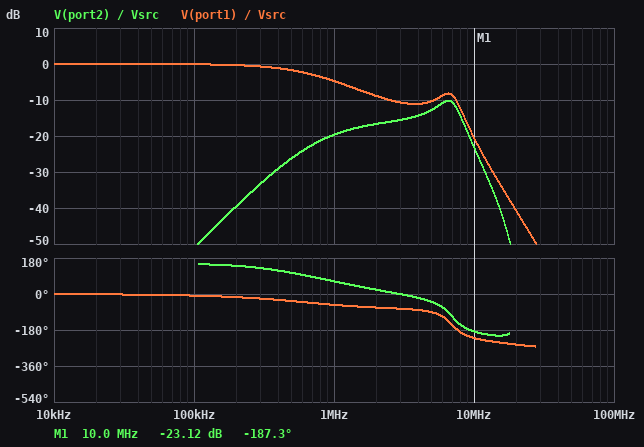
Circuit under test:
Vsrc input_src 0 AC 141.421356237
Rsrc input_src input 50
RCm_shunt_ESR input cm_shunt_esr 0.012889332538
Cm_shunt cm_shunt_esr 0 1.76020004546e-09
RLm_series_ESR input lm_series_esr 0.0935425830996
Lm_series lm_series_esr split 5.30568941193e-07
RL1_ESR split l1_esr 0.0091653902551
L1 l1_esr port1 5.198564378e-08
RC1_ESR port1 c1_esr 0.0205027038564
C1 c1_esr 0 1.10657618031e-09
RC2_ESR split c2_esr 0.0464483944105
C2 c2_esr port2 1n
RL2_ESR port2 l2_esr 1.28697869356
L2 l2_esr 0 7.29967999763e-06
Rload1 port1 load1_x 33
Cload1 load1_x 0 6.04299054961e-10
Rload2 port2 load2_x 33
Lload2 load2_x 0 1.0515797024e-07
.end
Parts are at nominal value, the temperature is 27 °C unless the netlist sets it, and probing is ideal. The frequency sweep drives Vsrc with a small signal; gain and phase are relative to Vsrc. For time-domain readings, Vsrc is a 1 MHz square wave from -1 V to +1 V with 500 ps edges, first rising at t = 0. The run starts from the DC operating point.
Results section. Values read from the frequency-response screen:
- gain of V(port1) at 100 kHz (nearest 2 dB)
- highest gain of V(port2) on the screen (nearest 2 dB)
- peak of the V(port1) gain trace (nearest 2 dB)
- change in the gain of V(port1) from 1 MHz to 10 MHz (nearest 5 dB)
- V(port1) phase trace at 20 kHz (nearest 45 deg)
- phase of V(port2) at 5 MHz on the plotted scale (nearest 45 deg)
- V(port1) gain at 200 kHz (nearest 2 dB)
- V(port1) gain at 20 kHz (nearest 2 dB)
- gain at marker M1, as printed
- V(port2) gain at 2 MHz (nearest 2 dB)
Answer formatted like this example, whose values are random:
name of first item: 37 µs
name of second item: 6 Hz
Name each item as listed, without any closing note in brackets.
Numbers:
gain of V(port1) at 100 kHz: 0 dB
highest gain of V(port2) on the screen: -10 dB
peak of the V(port1) gain trace: 0 dB
change in the gain of V(port1) from 1 MHz to 10 MHz: -15 dB
V(port1) phase trace at 20 kHz: 0 deg
phase of V(port2) at 5 MHz on the plotted scale: -45 deg
V(port1) gain at 200 kHz: 0 dB
V(port1) gain at 20 kHz: 0 dB
gain at marker M1, as printed: -23.12 dB
V(port2) gain at 2 MHz: -16 dB
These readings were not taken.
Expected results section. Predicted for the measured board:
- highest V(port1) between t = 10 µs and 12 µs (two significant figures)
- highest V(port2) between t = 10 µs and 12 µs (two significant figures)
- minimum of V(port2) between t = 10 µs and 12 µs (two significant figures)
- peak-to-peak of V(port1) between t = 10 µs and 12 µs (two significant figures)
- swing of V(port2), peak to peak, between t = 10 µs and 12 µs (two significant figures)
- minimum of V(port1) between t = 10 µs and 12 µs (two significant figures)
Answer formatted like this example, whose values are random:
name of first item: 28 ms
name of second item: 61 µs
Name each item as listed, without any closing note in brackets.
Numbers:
highest V(port1) between t = 10 µs and 12 µs: 810 mV
highest V(port2) between t = 10 µs and 12 µs: 330 mV
minimum of V(port2) between t = 10 µs and 12 µs: -330 mV
peak-to-peak of V(port1) between t = 10 µs and 12 µs: 1.6 V
swing of V(port2), peak to peak, between t = 10 µs and 12 µs: 670 mV
minimum of V(port1) between t = 10 µs and 12 µs: -810 mV
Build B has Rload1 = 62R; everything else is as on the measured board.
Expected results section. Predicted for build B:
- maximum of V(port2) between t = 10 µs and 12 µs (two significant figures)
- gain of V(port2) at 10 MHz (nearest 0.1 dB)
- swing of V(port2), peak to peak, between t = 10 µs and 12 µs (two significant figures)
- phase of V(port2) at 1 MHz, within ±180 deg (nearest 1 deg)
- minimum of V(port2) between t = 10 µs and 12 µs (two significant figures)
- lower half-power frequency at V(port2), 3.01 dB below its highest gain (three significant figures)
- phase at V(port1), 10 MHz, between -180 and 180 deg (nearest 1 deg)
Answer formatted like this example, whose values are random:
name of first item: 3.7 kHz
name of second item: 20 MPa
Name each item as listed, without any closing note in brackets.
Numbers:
maximum of V(port2) between t = 10 µs and 12 µs: 340 mV
gain of V(port2) at 10 MHz: -21.4 dB
swing of V(port2), peak to peak, between t = 10 µs and 12 µs: 680 mV
phase of V(port2) at 1 MHz, within ±180 deg: 64 deg
minimum of V(port2) between t = 10 µs and 12 µs: -340 mV
lower half-power frequency at V(port2), 3.01 dB below its highest gain: 4.71 MHz
phase at V(port1), 10 MHz, between -180 and 180 deg: 142 deg
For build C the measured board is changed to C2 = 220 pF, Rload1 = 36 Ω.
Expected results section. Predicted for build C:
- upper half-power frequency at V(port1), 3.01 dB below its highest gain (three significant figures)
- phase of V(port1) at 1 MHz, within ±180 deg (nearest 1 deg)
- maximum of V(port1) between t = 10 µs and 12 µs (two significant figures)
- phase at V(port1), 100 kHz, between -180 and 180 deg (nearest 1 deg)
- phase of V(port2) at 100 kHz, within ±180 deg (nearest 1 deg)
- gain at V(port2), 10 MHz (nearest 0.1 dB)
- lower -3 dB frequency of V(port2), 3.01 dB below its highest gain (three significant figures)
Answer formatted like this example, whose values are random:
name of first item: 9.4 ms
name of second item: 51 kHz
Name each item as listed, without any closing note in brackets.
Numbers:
upper half-power frequency at V(port1), 3.01 dB below its highest gain: 888 kHz
phase of V(port1) at 1 MHz, within ±180 deg: -49 deg
maximum of V(port1) between t = 10 µs and 12 µs: 890 mV
phase at V(port1), 100 kHz, between -180 and 180 deg: -7 deg
phase of V(port2) at 100 kHz, within ±180 deg: 150 deg
gain at V(port2), 10 MHz: -28.9 dB
lower -3 dB frequency of V(port2), 3.01 dB below its highest gain: 6.06 MHz
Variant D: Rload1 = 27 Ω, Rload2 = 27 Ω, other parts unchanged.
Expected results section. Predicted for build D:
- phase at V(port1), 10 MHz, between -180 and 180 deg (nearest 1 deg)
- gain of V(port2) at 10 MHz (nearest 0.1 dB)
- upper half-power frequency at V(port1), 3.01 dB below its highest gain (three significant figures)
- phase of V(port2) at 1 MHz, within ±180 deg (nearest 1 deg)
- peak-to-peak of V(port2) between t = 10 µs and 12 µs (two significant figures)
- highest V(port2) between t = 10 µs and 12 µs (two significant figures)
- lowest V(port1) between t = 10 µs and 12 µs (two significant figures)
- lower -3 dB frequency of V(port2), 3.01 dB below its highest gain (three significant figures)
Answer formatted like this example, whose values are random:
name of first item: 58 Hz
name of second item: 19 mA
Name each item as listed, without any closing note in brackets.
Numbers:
phase at V(port1), 10 MHz, between -180 and 180 deg: 139 deg
gain of V(port2) at 10 MHz: -24.2 dB
upper half-power frequency at V(port1), 3.01 dB below its highest gain: 714 kHz
phase of V(port2) at 1 MHz, within ±180 deg: 59 deg
peak-to-peak of V(port2) between t = 10 µs and 12 µs: 580 mV
highest V(port2) between t = 10 µs and 12 µs: 290 mV
lowest V(port1) between t = 10 µs and 12 µs: -810 mV
lower -3 dB frequency of V(port2), 3.01 dB below its highest gain: 4.98 MHz
